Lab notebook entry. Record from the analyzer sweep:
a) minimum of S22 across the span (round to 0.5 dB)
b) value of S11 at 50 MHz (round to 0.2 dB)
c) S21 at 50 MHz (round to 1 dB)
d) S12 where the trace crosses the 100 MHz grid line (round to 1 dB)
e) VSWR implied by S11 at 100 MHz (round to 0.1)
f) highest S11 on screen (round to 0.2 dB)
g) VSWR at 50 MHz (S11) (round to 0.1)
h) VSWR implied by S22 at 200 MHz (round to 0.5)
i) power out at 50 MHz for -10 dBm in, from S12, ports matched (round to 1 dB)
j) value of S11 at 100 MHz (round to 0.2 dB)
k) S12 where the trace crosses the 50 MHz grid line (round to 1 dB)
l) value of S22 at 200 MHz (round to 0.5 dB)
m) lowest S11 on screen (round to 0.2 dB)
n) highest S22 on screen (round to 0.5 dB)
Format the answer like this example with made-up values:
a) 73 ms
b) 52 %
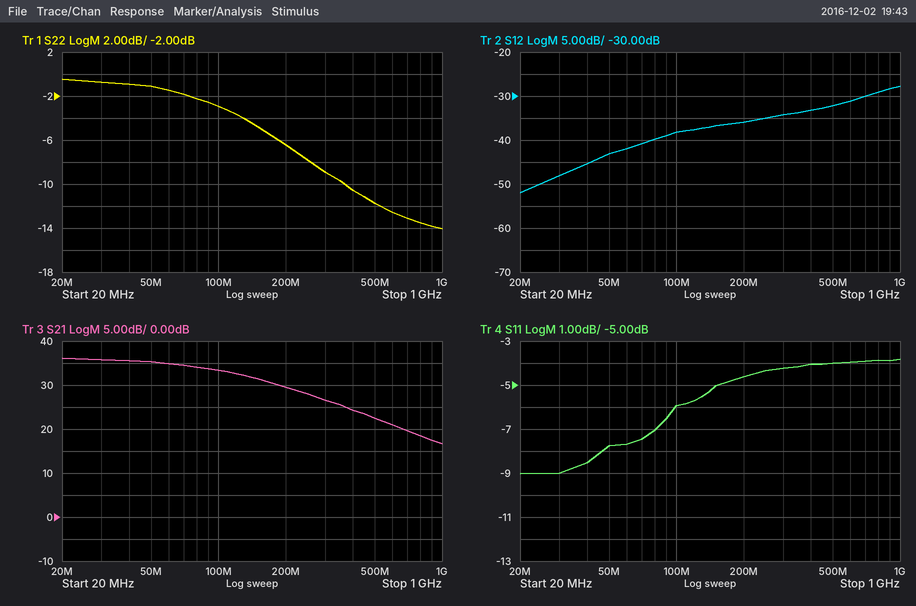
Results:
a) -14.0 dB
b) -7.8 dB
c) 35 dB
d) -38 dB
e) 3.0
f) -3.8 dB
g) 2.4
h) 3.0
i) -53 dBm
j) -6.0 dB
k) -43 dB
l) -6.5 dB
m) -9.0 dB
n) -0.5 dB
